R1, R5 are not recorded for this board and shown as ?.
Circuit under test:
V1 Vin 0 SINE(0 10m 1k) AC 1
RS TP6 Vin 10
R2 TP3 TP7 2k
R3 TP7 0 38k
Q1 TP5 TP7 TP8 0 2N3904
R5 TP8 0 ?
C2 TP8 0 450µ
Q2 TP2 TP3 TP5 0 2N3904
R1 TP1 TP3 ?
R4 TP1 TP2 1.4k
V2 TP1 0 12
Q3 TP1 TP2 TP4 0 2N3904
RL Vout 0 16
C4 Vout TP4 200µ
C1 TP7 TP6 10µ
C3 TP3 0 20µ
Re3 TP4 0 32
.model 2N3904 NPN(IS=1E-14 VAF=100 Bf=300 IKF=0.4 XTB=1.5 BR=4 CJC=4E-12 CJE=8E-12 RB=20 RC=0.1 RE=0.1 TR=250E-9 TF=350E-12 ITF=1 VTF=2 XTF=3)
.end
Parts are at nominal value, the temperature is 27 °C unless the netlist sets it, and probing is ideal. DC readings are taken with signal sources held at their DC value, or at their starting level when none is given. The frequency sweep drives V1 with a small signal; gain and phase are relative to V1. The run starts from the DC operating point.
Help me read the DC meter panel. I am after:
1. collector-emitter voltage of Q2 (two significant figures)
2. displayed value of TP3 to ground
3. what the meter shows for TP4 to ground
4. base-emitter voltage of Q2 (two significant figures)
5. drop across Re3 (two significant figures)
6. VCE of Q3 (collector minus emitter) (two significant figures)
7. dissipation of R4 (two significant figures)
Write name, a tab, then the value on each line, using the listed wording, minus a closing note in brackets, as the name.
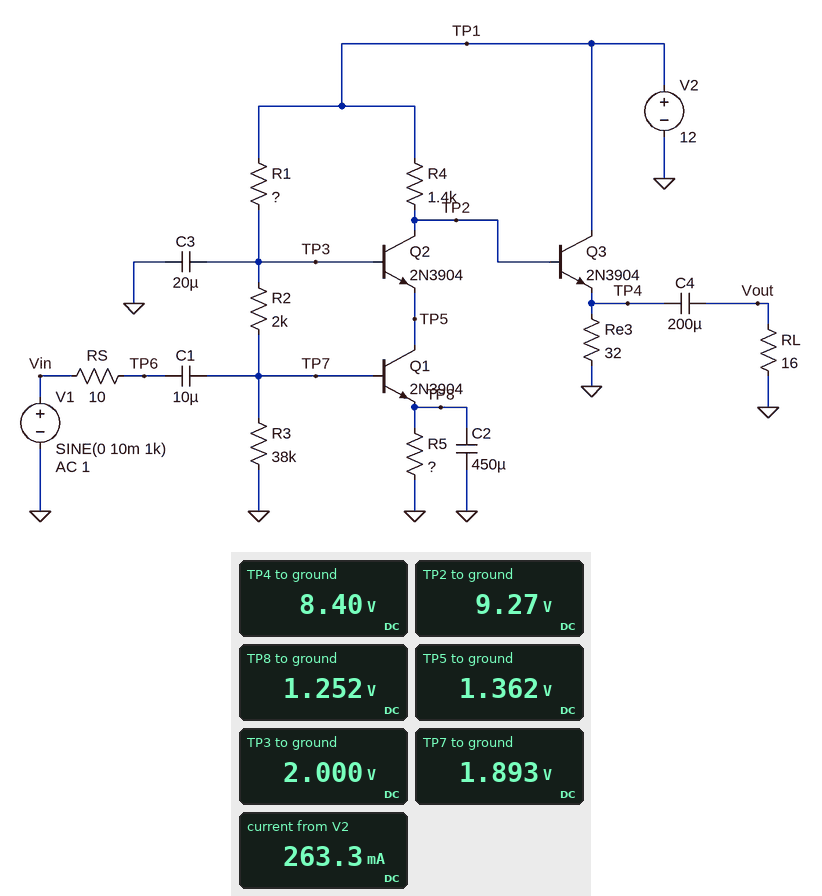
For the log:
collector-emitter voltage of Q2	7.9 V
displayed value of TP3 to ground	2.000 V
what the meter shows for TP4 to ground	8.40 V
base-emitter voltage of Q2	640 mV
drop across Re3	8.4 V
VCE of Q3 (collector minus emitter)	3.6 V
dissipation of R4	5.3 mW
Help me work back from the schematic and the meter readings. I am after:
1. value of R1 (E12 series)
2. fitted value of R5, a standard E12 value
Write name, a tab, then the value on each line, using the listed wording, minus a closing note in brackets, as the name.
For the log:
value of R1	180 kΩ
fitted value of R5, a standard E12 value	2.2 kΩ
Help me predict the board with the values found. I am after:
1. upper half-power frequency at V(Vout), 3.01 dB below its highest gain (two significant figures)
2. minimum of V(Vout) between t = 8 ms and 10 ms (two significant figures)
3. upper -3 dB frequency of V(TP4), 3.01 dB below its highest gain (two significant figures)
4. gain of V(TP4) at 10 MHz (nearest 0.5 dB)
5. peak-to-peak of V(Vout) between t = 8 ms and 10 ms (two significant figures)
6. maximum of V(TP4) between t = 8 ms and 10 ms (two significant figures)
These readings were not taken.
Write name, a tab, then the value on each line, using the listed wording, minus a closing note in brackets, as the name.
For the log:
upper half-power frequency at V(Vout), 3.01 dB below its highest gain	4.3 MHz
minimum of V(Vout) between t = 8 ms and 10 ms	-160 mV
upper -3 dB frequency of V(TP4), 3.01 dB below its highest gain	3.3 MHz
gain of V(TP4) at 10 MHz	14.5 dB
peak-to-peak of V(Vout) between t = 8 ms and 10 ms	290 mV
maximum of V(TP4) between t = 8 ms and 10 ms	8.5 V
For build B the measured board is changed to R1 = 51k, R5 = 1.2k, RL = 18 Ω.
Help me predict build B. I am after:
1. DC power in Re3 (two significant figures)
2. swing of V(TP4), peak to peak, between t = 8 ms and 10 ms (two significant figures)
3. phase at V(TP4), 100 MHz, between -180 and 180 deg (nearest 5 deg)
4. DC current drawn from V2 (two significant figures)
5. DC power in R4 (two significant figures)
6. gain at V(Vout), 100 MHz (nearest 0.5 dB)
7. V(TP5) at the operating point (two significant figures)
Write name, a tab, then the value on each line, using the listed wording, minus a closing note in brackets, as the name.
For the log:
DC power in Re3	980 mW
swing of V(TP4), peak to peak, between t = 8 ms and 10 ms	1.9 V
phase at V(TP4), 100 MHz, between -180 and 180 deg	30 deg
DC current drawn from V2	180 mA
DC power in R4	22 mW
gain at V(Vout), 100 MHz	9.5 dB
V(TP5) at the operating point	4.1 V
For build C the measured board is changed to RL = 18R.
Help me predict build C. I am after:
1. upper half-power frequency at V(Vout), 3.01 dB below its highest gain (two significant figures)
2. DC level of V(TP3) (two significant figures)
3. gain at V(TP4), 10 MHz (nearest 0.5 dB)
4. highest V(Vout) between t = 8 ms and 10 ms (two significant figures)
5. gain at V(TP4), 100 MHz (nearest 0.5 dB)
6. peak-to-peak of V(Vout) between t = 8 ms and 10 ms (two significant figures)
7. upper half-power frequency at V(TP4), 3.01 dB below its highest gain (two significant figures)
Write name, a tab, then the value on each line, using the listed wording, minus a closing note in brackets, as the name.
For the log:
upper half-power frequency at V(Vout), 3.01 dB below its highest gain	4.4 MHz
DC level of V(TP3)	2.0 V
gain at V(TP4), 10 MHz	15.0 dB
highest V(Vout) between t = 8 ms and 10 ms	140 mV
gain at V(TP4), 100 MHz	-11.0 dB
peak-to-peak of V(Vout) between t = 8 ms and 10 ms	300 mV
upper half-power frequency at V(TP4), 3.01 dB below its highest gain	3.7 MHz
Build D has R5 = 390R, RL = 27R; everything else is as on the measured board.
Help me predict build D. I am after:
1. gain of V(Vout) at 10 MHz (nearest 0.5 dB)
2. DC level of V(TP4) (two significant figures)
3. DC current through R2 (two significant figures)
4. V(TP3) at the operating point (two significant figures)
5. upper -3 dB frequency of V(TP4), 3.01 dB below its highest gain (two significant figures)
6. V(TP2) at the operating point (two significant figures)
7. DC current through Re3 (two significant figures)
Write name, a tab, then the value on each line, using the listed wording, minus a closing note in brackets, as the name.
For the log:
gain of V(Vout) at 10 MHz	24.5 dB
DC level of V(TP4)	7.0 V
DC current through R2	52 µA
V(TP3) at the operating point	1.5 V
upper -3 dB frequency of V(TP4), 3.01 dB below its highest gain	4.1 MHz
V(TP2) at the operating point	7.8 V
DC current through Re3	220 mA
